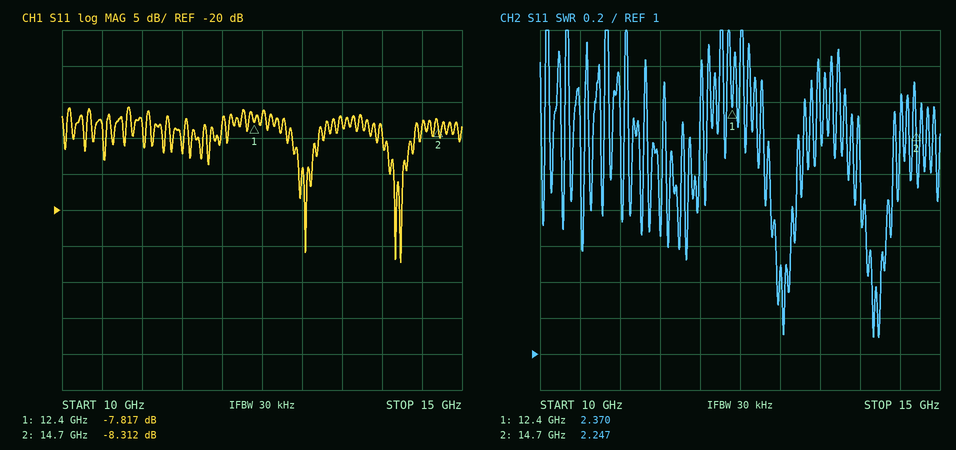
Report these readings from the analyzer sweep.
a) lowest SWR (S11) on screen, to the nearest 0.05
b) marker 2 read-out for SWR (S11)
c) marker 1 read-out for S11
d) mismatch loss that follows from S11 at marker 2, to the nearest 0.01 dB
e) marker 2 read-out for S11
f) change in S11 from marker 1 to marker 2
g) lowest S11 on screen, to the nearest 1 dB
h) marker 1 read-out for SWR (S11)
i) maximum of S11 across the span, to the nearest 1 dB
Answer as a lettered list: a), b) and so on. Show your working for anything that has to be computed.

a) 1.10
b) 2.247
c) -7.817 dB
d) −10 log10(1 − 10^(-8.312/10)) ≈ 0.69 dB
e) -8.312 dB
f) -8.312 − (-7.817) = -0.495 dB
g) -27 dB
h) 2.370
i) -6 dB
